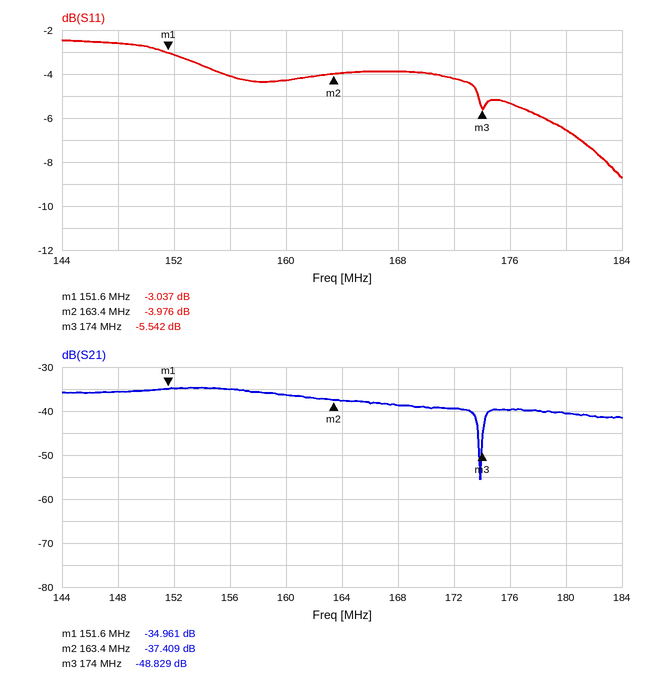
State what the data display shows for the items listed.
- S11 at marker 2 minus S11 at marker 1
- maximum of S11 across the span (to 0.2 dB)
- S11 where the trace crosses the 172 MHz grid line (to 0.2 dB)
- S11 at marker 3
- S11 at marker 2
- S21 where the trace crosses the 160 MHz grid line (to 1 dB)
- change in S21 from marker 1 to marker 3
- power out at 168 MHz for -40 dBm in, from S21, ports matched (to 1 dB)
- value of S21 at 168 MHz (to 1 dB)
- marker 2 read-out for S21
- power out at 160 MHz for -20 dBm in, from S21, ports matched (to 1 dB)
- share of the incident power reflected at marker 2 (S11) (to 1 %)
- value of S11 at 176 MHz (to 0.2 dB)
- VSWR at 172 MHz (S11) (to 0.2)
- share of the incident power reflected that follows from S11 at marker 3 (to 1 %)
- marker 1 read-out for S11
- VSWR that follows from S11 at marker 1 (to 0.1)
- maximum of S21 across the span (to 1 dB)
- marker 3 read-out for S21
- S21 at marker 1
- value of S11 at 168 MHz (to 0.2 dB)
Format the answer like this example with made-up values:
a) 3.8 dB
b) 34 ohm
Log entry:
a) -0.939 dB
b) -2.4 dB
c) -4.2 dB
d) -5.542 dB
e) -3.976 dB
f) -36 dB
g) -13.868 dB
h) -79 dBm
i) -39 dB
j) -37.409 dB
k) -56 dBm
l) 40 %
m) -5.4 dB
n) 4.2
o) 28 %
p) -3.037 dB
q) 5.8
r) -35 dB
s) -48.829 dB
t) -34.961 dB
u) -3.8 dB
